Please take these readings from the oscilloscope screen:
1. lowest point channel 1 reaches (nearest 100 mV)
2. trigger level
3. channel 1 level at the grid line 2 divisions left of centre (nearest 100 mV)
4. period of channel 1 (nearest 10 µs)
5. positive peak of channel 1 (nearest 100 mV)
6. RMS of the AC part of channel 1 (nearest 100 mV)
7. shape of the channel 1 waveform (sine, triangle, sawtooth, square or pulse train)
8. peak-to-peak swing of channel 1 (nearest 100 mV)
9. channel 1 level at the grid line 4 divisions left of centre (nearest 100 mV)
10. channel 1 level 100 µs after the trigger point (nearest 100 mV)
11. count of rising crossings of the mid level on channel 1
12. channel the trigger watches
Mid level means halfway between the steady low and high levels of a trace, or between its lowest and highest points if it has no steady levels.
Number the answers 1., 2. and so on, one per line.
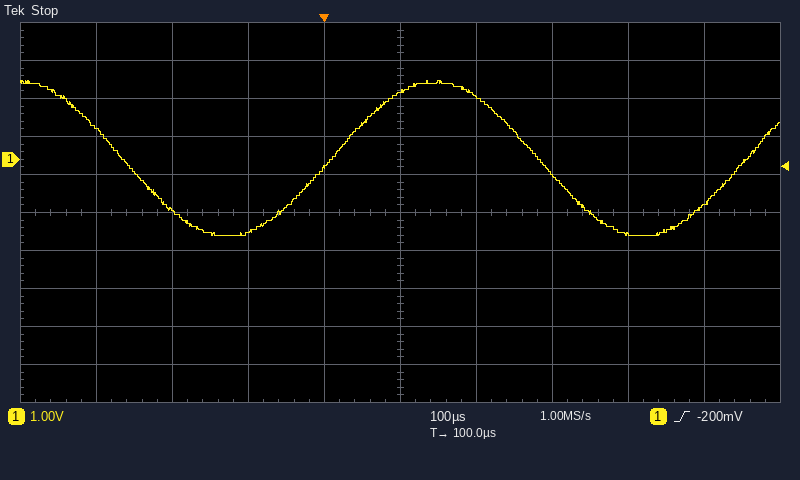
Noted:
1. -2.0 V
2. -200 mV
3. -1.9 V
4. 550 µs
5. 2.1 V
6. 1.4 V
7. sine
8. 4.1 V
9. 800 mV
10. 1.8 V
11. 2
12. channel 1
